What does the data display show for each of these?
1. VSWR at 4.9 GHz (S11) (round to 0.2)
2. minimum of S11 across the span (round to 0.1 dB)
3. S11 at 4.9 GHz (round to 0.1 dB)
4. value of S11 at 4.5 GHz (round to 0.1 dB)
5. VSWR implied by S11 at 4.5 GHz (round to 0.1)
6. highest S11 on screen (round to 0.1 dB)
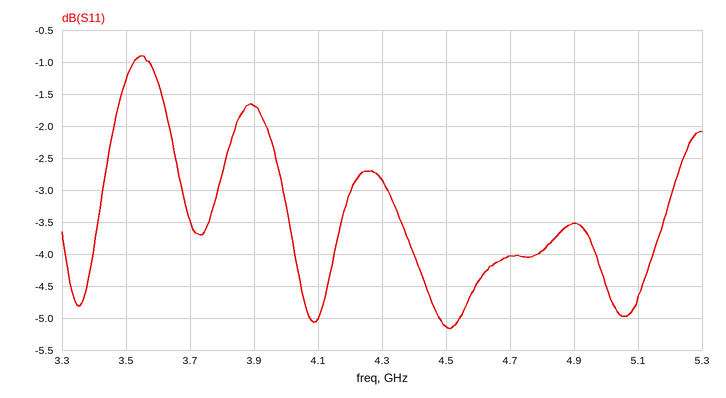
5.0
-5.2 dB
-3.5 dB
-5.1 dB
3.5
-0.9 dB
